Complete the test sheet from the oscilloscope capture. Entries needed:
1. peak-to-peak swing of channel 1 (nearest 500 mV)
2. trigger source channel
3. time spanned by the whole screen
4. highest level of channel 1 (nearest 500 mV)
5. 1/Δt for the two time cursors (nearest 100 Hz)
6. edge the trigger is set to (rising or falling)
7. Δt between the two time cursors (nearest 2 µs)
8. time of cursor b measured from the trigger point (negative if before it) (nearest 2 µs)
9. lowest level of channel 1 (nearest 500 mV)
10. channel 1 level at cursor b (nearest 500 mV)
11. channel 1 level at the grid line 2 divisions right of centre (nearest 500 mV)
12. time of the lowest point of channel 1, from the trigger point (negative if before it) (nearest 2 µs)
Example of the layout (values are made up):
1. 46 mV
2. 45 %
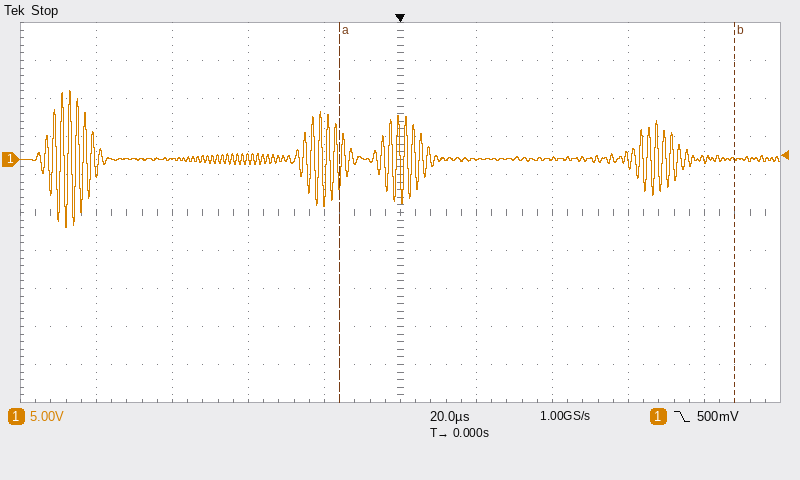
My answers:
1. 18.0 V
2. channel 1
3. 200 µs
4. 9.0 V
5. 9.6 kHz
6. falling
7. 104 µs
8. +88 µs
9. -9.0 V
10. 0.0 V
11. 0.0 V
12. -88 µs
